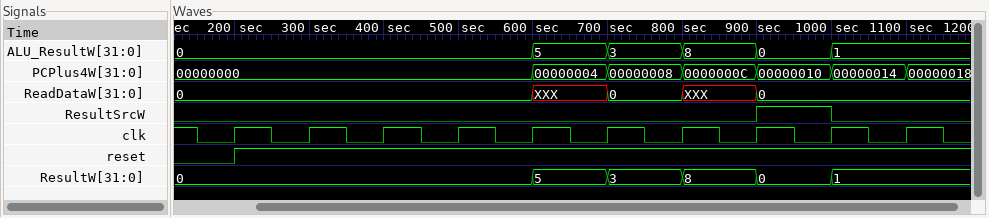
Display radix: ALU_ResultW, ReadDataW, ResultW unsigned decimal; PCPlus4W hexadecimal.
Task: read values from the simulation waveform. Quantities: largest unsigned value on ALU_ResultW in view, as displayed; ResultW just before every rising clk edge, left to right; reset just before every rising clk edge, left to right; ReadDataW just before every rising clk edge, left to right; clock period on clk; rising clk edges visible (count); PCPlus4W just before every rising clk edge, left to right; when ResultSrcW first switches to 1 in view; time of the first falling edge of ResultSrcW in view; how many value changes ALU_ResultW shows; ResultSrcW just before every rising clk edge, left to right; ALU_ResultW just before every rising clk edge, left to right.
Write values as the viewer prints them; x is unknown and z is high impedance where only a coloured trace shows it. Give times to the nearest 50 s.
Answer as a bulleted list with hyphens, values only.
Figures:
- 8
- 0, 0, 0, 0, 0, 5, 3, 8, 0, 1
- 0 1 1 1 1 1 1 1 1 1
- 0, 0, 0, 0, 0, XXX, 0, XXX, 0, 0
- 100 s
- 10
- 00000000, 00000000, 00000000, 00000000, 00000000, 00000004, 00000008, 0000000C, 00000010, 00000014
- 900 s
- 1000 s
- 5
- 0 0 0 0 0 0 0 0 1 0
- 0, 0, 0, 0, 0, 5, 3, 8, 0, 1
